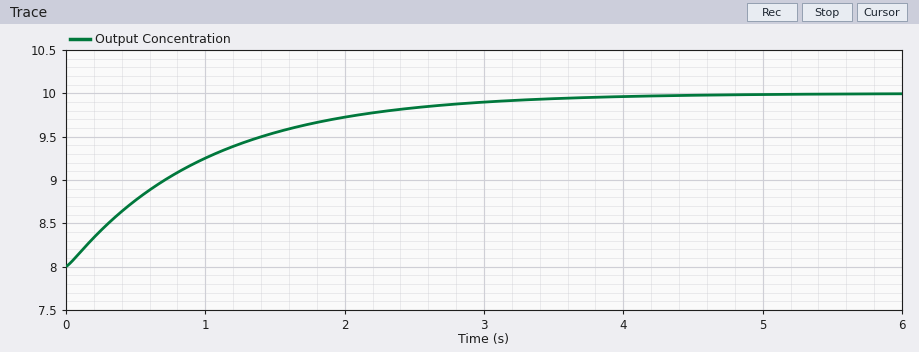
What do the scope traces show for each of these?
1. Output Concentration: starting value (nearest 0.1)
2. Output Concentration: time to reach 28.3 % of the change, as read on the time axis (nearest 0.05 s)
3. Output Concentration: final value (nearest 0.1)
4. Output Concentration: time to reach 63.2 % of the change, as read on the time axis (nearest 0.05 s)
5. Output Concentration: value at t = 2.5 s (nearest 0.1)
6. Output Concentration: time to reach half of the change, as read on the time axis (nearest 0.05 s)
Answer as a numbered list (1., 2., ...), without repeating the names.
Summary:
1. 8.0
2. 0.35 s
3. 10.0
4. 1.00 s
5. 9.8
6. 0.70 s
